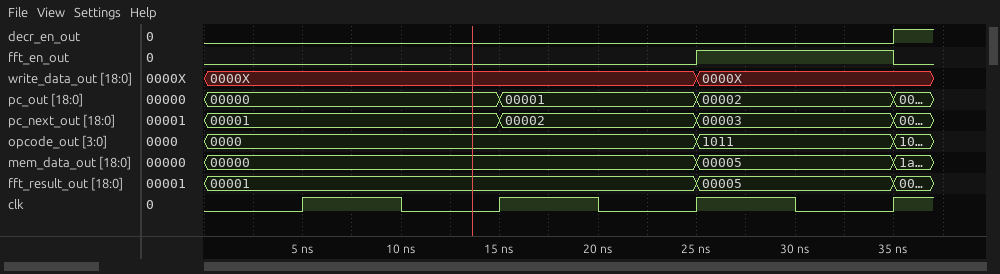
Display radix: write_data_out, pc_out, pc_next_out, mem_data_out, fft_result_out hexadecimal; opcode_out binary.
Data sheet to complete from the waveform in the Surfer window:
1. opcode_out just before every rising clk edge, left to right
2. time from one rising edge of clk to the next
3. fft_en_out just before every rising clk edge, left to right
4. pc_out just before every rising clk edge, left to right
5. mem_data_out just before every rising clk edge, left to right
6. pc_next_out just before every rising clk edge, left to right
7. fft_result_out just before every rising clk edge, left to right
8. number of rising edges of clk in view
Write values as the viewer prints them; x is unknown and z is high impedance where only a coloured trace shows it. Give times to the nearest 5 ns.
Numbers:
0000, 0000, 0000, 1011
10 ns
0 0 0 1
00000, 00000, 00001, 00002
00000, 00000, 00000, 00005
00001, 00001, 00002, 00003
00001, 00001, 00001, 00005
4
